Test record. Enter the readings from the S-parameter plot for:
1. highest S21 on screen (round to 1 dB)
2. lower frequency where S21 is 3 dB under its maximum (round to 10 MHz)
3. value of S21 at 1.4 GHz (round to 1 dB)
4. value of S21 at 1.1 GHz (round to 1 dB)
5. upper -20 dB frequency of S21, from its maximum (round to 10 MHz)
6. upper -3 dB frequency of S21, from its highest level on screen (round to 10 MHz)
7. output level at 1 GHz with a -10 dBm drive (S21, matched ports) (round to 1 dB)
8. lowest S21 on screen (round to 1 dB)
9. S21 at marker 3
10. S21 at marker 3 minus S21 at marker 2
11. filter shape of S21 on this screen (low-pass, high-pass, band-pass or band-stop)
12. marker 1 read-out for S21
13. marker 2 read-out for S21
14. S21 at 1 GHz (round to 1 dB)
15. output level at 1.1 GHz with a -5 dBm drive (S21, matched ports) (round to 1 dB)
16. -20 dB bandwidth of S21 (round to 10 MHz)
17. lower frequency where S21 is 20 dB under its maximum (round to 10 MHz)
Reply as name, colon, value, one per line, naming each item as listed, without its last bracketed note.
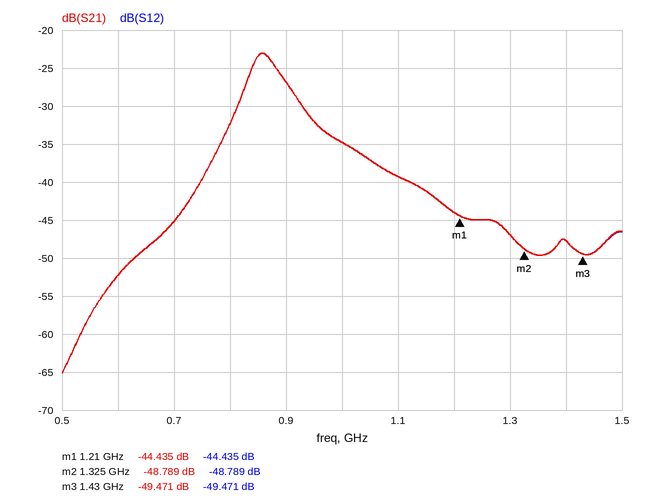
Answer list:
highest S21 on screen: -23 dB
lower frequency where S21 is 3 dB under its maximum: 830 MHz
value of S21 at 1.4 GHz: -48 dB
value of S21 at 1.1 GHz: -39 dB
upper -20 dB frequency of S21, from its maximum: 1.18 GHz
upper -3 dB frequency of S21, from its highest level on screen: 890 MHz
output level at 1 GHz with a -10 dBm drive (S21, matched ports): -45 dBm
lowest S21 on screen: -65 dB
S21 at marker 3: -49.471 dB
S21 at marker 3 minus S21 at marker 2: -0.682 dB
filter shape of S21 on this screen: band-pass
marker 1 read-out for S21: -44.435 dB
marker 2 read-out for S21: -48.789 dB
S21 at 1 GHz: -35 dB
output level at 1.1 GHz with a -5 dBm drive (S21, matched ports): -44 dBm
-20 dB bandwidth of S21: 460 MHz
lower frequency where S21 is 20 dB under its maximum: 720 MHz
